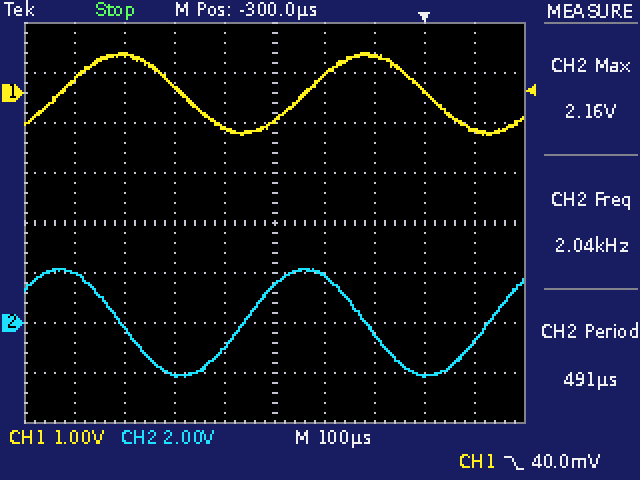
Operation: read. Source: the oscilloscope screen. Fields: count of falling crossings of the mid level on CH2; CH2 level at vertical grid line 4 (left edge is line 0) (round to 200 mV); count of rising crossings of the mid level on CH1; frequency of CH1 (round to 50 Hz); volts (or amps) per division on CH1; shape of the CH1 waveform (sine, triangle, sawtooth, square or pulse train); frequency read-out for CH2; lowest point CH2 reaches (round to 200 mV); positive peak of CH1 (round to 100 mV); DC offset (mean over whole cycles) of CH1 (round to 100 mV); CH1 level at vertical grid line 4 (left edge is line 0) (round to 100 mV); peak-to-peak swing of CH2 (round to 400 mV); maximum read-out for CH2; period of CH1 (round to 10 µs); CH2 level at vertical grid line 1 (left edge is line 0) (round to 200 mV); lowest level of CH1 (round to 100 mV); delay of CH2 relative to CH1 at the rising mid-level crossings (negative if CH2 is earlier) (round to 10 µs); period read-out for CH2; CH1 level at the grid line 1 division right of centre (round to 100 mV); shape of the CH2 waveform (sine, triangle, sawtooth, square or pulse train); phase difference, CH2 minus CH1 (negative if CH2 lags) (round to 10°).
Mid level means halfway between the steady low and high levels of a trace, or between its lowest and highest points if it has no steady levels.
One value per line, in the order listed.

2
-1.0 V
2
2.05 kHz
1 V
sine
2.04 kHz
-2.2 V
800 mV
0.0 V
-700 mV
4.4 V
2.16 V
490 µs
2.0 V
-800 mV
-120 µs
491 µs
400 mV
sine
+90°
